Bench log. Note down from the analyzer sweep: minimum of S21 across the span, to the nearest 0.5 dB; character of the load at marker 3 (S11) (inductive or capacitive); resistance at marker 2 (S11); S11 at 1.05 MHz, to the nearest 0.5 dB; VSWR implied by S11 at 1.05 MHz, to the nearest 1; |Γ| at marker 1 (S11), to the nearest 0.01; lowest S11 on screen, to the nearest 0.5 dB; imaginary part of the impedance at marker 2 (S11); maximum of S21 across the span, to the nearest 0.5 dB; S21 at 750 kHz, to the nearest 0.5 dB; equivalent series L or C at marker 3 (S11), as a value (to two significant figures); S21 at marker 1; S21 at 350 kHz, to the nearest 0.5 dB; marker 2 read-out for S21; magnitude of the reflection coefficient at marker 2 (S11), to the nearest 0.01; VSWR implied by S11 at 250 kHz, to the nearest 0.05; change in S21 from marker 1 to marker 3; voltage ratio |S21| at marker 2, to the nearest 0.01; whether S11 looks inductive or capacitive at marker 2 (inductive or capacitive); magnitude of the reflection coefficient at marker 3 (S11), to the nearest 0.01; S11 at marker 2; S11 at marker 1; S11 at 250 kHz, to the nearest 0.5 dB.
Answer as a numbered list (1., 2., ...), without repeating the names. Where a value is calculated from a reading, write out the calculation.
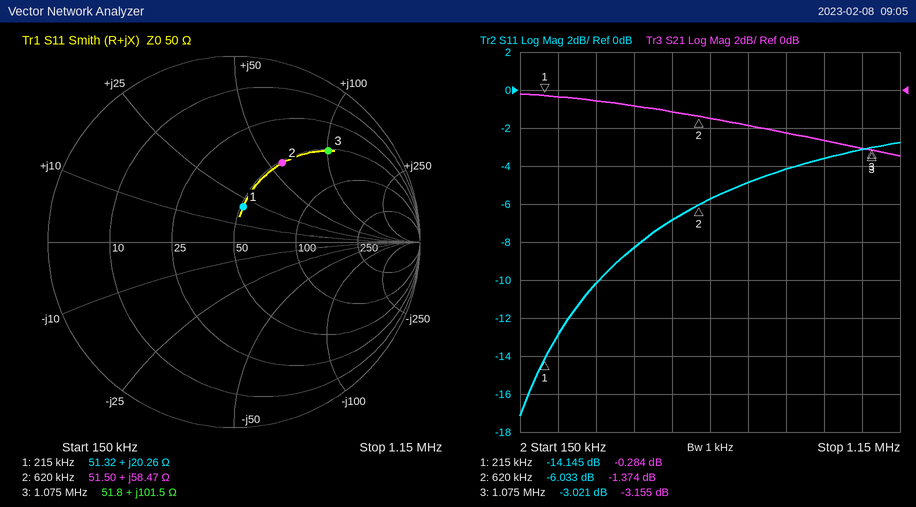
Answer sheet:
1. -3.5 dB
2. inductive
3. 51.50 Ω
4. -3.0 dB
5. |Γ| = 10^(-3/20) = 0.7079; VSWR = (1 + 0.7079)/(1 − 0.7079) ≈ 6
6. 0.20
7. -17.0 dB
8. +58.47 Ω
9. 0.0 dB
10. -2.0 dB
11. L = 101.5 Ω/(2π × 1.075 MHz) ≈ 15 µH
12. -0.284 dB
13. -0.5 dB
14. -1.374 dB
15. 0.50
16. |Γ| = 10^(-13/20) = 0.2239; VSWR = (1 + 0.2239)/(1 − 0.2239) ≈ 1.58, so 1.60 to the nearest 0.05
17. -3.155 − (-0.284) = -2.871 dB
18. 10^(-1.374/20) ≈ 0.85
19. inductive
20. 0.71
21. -6.033 dB
22. -14.145 dB
23. -13.0 dB
